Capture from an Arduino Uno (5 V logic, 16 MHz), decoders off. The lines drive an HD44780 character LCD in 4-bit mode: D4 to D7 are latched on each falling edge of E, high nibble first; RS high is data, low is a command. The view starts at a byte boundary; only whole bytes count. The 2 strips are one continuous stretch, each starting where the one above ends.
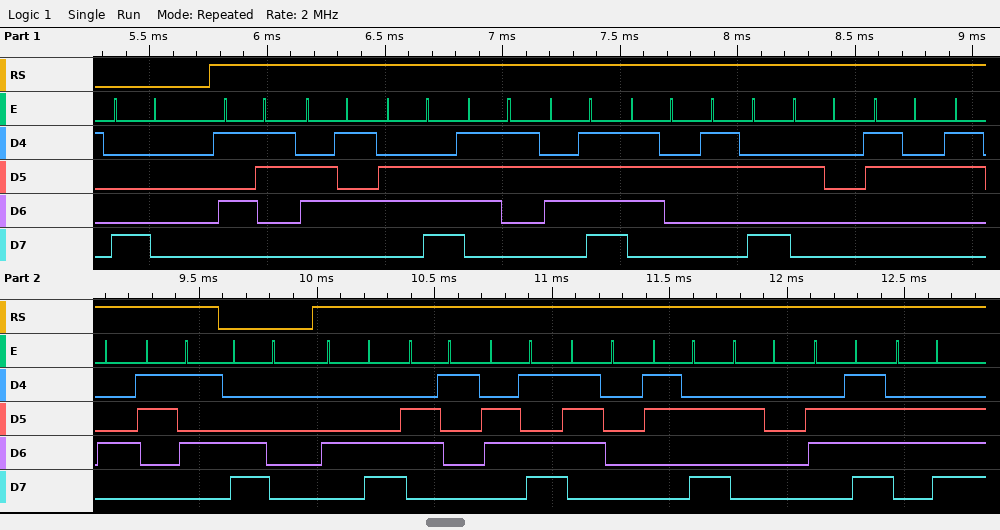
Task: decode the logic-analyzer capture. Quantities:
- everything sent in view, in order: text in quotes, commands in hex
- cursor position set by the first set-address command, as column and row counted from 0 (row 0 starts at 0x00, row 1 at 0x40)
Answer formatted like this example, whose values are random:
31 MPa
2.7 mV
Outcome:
0x80 "Sensor: 245" 0xC0 "Lamp: on"
column 0, row 0
